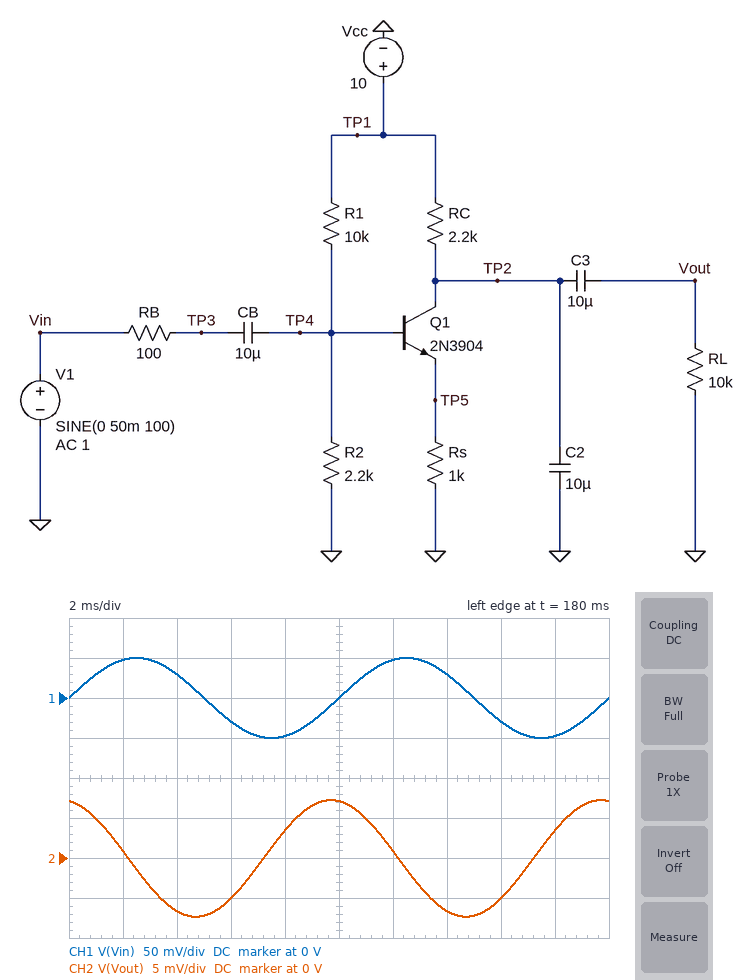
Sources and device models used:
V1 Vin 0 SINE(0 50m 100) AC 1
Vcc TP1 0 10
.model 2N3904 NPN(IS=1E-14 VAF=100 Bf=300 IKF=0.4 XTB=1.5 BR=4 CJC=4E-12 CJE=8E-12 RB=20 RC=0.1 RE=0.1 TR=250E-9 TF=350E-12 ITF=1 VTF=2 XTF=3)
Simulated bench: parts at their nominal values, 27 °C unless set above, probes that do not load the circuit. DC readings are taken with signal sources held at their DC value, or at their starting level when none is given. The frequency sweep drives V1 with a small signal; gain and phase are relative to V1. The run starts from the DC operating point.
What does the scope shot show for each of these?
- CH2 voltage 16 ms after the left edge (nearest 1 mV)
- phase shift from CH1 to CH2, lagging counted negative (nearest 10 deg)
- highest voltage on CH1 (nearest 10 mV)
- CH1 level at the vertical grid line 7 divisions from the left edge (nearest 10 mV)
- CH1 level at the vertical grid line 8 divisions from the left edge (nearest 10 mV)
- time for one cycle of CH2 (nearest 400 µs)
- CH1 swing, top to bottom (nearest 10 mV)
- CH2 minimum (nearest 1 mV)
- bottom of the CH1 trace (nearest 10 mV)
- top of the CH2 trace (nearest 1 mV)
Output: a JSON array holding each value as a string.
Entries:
["-5 mV", "100 deg", "50 mV", "30 mV", "-30 mV", "10.0 ms", "100 mV", "-7 mV", "-50 mV", "7 mV"]
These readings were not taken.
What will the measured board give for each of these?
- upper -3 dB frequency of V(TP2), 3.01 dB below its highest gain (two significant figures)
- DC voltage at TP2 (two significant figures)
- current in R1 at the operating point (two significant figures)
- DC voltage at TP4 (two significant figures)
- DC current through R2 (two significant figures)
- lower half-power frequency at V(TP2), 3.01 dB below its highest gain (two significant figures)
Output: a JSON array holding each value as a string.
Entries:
["21 Hz", "7.5 V", "820 µA", "1.8 V", "820 µA", "3.5 Hz"]
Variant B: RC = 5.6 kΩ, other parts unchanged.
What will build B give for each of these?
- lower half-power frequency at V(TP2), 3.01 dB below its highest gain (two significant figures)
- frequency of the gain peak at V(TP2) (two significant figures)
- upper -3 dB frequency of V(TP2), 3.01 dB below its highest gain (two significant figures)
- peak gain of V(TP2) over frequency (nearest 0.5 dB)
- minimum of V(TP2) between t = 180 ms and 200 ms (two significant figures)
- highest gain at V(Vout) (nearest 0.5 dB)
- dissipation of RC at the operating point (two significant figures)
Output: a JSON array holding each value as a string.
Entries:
["2.3 Hz", "6.3 Hz", "16 Hz", "1.0 dB", "3.6 V", "0.5 dB", "7.2 mW"]
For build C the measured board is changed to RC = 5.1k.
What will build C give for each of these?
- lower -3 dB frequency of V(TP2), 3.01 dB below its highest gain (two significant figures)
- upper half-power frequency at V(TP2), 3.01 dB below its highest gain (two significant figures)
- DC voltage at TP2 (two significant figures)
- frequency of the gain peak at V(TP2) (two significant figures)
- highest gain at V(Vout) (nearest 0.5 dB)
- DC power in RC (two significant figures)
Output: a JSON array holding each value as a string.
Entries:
["2.4 Hz", "16 Hz", "4.2 V", "6.5 Hz", "0.5 dB", "6.6 mW"]
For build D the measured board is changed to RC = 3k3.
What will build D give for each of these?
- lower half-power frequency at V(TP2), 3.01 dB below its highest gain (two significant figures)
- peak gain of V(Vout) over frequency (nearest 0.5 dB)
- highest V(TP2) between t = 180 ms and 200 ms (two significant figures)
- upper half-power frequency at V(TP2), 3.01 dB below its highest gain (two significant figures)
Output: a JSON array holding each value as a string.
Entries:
["2.9 Hz", "-0.5 dB", "6.3 V", "18 Hz"]
